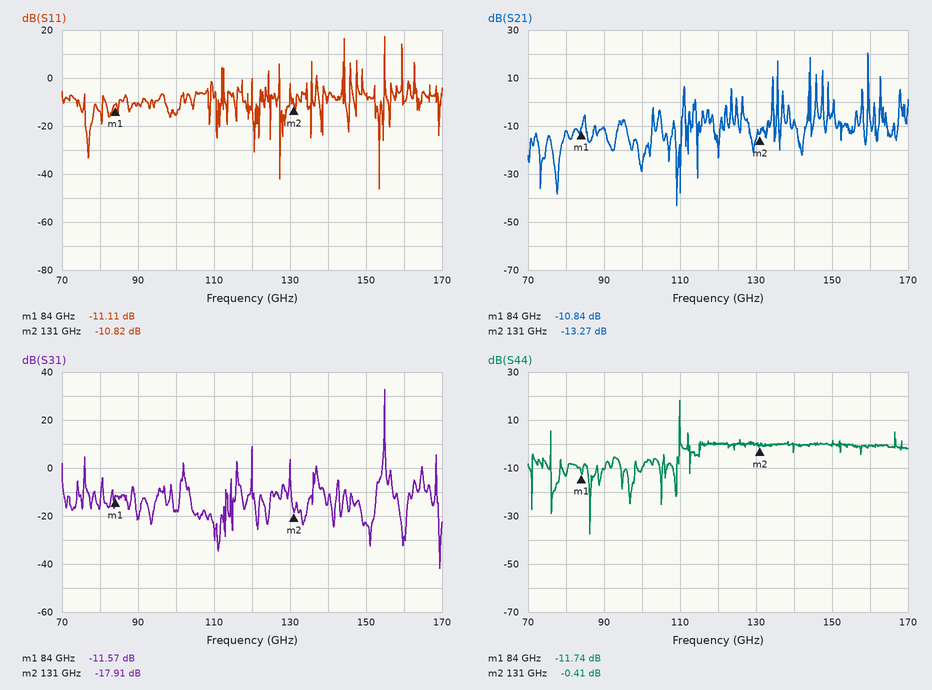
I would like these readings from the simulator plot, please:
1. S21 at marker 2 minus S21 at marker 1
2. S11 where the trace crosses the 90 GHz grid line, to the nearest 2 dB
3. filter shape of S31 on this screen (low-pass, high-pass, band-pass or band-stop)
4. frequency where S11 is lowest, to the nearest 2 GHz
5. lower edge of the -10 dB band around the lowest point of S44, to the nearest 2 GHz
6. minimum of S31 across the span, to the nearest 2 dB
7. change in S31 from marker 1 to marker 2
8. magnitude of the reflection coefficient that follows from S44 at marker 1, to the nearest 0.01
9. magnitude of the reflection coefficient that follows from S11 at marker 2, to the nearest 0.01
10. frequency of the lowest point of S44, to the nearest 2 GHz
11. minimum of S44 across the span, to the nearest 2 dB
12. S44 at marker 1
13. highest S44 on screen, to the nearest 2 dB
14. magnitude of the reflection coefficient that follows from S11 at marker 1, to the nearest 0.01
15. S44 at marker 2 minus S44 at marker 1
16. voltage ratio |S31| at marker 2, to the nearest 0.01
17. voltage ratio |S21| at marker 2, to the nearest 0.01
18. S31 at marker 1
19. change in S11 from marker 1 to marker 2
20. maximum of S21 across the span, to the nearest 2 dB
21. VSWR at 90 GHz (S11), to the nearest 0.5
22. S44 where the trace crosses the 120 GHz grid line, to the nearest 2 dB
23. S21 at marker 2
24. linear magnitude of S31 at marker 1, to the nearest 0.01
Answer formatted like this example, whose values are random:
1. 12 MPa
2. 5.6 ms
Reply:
1. -2.43 dB
2. -10 dB
3. band-pass
4. 154 GHz
5. 86 GHz
6. -42 dB
7. -6.34 dB
8. 0.26
9. 0.29
10. 86 GHz
11. -38 dB
12. -11.74 dB
13. 18 dB
14. 0.28
15. 11.33 dB
16. 0.13
17. 0.22
18. -11.57 dB
19. 0.29 dB
20. 20 dB
21. 2.0
22. 0 dB
23. -13.27 dB
24. 0.26
